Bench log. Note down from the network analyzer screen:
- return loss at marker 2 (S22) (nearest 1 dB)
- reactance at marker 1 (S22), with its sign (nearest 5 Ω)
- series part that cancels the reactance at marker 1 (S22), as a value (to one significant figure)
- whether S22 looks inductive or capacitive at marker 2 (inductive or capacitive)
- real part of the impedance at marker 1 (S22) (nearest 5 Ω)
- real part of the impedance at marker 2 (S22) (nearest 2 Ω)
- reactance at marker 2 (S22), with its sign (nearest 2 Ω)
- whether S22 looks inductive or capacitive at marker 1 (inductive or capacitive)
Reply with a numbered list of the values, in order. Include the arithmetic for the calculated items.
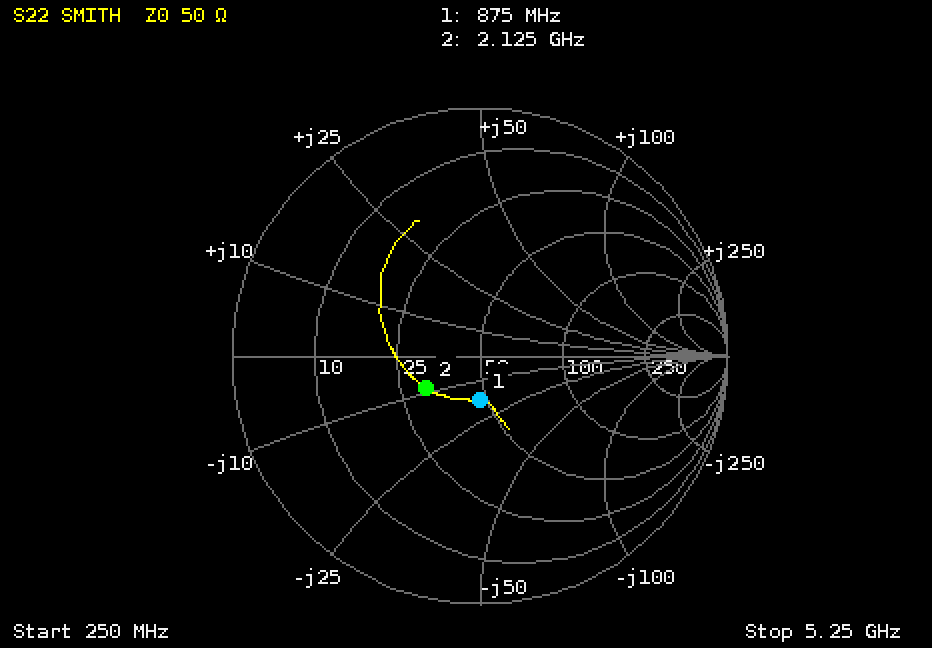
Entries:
1. 12 dB
2. -15 Ω
3. L = 15 Ω/(2π × 875 MHz) ≈ 3 nH
4. capacitive
5. 45 Ω
6. 32 Ω
7. -8 Ω
8. capacitive
